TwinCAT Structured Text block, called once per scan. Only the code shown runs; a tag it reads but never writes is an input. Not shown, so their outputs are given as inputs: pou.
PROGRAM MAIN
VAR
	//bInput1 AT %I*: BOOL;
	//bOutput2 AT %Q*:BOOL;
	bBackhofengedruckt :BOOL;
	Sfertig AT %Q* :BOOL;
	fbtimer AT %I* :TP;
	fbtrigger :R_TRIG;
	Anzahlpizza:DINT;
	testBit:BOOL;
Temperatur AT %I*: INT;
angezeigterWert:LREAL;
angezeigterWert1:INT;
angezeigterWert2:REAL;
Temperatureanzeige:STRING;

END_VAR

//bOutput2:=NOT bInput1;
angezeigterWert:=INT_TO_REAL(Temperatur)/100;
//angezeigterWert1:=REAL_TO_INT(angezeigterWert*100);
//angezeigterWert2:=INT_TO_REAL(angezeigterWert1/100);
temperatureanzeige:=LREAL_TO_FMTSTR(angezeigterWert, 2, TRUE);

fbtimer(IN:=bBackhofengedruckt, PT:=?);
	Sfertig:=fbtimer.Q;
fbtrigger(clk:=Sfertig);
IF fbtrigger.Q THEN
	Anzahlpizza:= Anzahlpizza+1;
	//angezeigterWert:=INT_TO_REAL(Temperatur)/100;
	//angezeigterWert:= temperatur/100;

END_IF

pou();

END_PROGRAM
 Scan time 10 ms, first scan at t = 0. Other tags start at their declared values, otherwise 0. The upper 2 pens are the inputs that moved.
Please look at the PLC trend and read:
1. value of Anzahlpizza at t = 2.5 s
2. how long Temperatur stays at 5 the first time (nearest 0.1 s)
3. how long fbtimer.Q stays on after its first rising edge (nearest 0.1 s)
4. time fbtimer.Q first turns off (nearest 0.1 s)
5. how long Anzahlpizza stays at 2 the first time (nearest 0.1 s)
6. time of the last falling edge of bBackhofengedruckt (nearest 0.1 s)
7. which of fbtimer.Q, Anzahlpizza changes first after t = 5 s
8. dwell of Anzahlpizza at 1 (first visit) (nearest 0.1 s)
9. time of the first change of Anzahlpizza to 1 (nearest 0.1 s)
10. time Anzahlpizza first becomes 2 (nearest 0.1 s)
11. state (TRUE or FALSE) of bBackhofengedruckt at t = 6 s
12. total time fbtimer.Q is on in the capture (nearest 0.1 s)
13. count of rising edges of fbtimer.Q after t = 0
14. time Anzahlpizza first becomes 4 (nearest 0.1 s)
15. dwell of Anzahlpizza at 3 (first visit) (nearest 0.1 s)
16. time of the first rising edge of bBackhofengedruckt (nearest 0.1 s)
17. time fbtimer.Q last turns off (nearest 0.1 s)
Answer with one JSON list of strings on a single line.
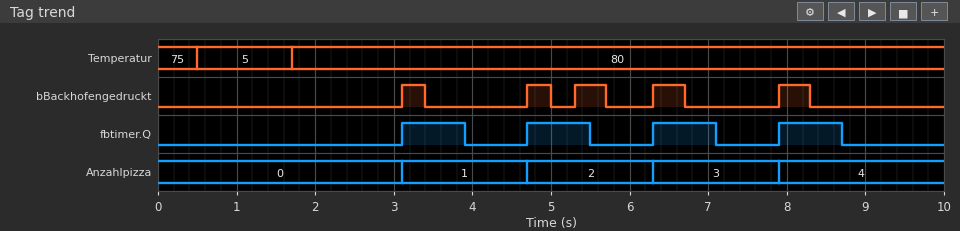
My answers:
["0", "1.2 s", "0.8 s", "3.9 s", "1.6 s", "8.3 s", "fbtimer.Q", "1.6 s", "3.1 s", "4.7 s", "FALSE", "3.2 s", "4", "7.9 s", "1.6 s", "3.1 s", "8.7 s"]
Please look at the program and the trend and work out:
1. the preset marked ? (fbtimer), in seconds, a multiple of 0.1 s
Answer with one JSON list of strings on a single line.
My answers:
["0.8 s"]
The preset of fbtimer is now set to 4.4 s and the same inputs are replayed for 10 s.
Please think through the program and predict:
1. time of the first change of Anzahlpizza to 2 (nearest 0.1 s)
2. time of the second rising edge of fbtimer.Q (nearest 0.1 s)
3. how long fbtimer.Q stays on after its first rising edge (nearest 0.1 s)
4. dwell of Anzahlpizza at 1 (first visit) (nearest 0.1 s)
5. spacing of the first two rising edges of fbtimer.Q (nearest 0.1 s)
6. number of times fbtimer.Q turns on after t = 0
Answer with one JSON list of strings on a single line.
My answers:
["7.9 s", "7.9 s", "4.4 s", "4.8 s", "4.8 s", "2"]
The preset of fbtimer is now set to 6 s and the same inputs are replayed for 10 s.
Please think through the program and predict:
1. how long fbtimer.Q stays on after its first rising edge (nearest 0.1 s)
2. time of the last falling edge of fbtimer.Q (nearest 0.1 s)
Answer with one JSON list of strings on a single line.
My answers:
["6.0 s", "9.1 s"]
